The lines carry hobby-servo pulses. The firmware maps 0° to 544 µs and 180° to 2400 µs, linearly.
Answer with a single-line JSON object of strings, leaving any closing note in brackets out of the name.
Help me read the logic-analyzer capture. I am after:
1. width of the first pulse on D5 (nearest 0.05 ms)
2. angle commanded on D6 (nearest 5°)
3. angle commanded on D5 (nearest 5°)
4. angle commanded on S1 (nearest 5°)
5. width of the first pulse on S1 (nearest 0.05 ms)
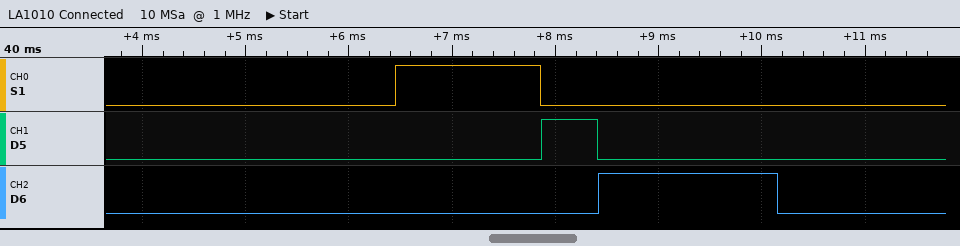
{"width of the first pulse on D5": "0.55 ms", "angle commanded on D6": "115°", "angle commanded on D5": "0°", "angle commanded on S1": "85°", "width of the first pulse on S1": "1.40 ms"}
